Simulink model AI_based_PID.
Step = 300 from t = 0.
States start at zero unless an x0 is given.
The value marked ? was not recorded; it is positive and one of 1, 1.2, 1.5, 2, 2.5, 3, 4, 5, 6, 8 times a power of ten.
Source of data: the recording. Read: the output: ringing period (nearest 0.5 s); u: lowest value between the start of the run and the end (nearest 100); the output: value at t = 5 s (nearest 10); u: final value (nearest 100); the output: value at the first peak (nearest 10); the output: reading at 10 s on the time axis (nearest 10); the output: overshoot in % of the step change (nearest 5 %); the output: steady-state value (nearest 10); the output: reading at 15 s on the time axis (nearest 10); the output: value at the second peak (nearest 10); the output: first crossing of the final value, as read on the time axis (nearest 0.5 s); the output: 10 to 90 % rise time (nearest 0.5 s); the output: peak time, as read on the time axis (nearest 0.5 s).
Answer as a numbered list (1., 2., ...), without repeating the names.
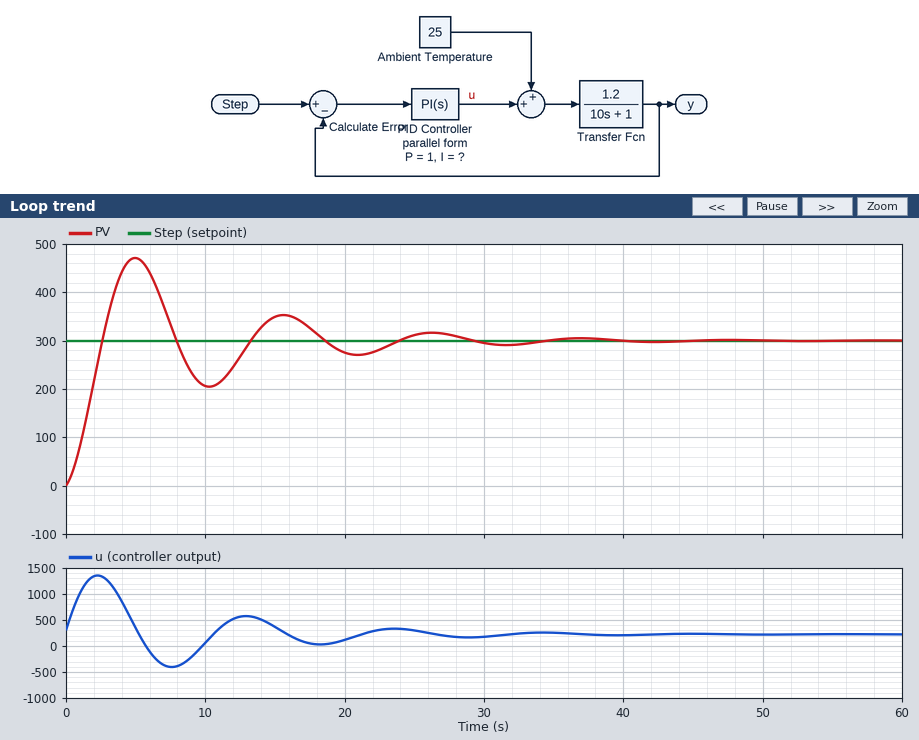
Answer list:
1. 10.5 s
2. -400
3. 470
4. 200
5. 470
6. 210
7. 55 %
8. 300
9. 350
10. 350
11. 2.5 s
12. 2.0 s
13. 5.0 s
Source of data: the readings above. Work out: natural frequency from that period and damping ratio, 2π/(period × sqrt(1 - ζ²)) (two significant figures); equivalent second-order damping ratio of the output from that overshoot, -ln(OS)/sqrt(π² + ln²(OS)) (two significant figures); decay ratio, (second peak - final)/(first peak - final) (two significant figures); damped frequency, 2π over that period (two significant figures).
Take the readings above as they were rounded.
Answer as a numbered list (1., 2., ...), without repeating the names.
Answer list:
1. 0.61 rad/s
2. 0.19
3. 0.29
4. 0.60 rad/s
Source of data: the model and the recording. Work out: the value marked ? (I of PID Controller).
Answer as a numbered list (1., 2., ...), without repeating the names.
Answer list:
1. 3
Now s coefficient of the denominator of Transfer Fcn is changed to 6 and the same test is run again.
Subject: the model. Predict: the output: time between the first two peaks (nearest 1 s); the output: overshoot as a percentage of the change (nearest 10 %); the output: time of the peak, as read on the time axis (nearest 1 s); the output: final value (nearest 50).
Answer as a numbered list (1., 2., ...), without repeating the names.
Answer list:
1. 8 s
2. 50 %
3. 4 s
4. 300
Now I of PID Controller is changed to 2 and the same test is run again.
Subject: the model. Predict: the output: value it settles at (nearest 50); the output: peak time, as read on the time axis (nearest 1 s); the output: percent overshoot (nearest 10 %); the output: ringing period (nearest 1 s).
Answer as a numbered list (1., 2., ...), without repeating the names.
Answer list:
1. 300
2. 6 s
3. 50 %
4. 13 s
